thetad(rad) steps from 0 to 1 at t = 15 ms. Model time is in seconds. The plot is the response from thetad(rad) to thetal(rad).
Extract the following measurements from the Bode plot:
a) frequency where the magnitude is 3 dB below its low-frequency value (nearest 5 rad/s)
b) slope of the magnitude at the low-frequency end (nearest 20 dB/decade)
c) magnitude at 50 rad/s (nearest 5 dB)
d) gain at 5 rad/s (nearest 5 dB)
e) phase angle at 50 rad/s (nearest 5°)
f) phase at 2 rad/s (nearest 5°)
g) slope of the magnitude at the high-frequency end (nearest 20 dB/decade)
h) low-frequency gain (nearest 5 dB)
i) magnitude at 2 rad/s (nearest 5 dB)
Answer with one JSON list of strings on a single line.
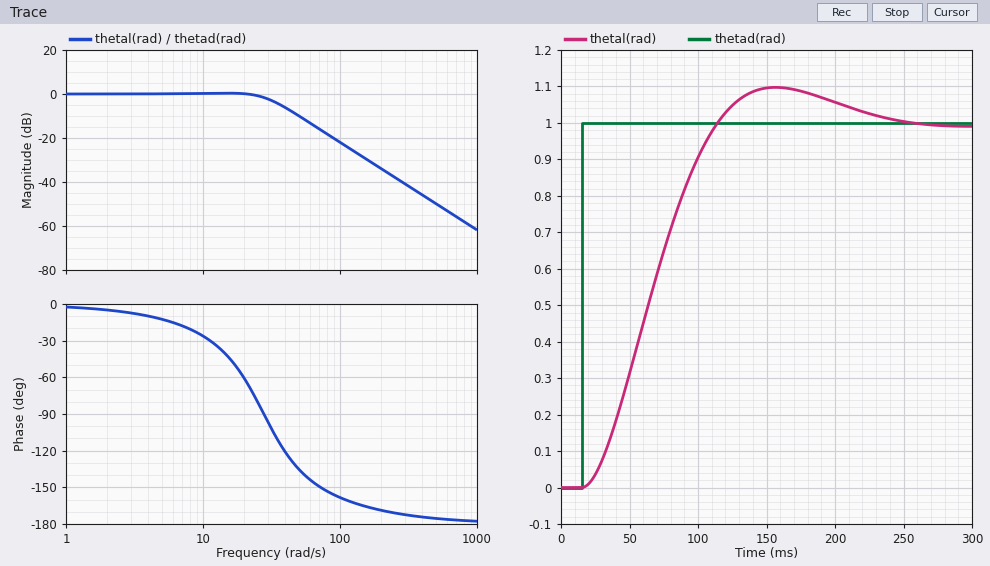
["30 rad/s", "0 dB/decade", "-10 dB", "0 dB", "-135°", "-5°", "-40 dB/decade", "0 dB", "0 dB"]
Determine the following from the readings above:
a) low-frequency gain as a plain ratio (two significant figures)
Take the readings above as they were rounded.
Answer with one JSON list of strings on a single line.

["1.0"]
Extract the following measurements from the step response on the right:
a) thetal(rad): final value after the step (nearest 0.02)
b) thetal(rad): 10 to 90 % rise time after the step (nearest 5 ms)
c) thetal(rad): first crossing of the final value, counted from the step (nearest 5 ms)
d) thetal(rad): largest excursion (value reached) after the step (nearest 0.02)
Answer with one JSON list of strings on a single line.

["1.00", "65 ms", "100 ms", "1.10"]
